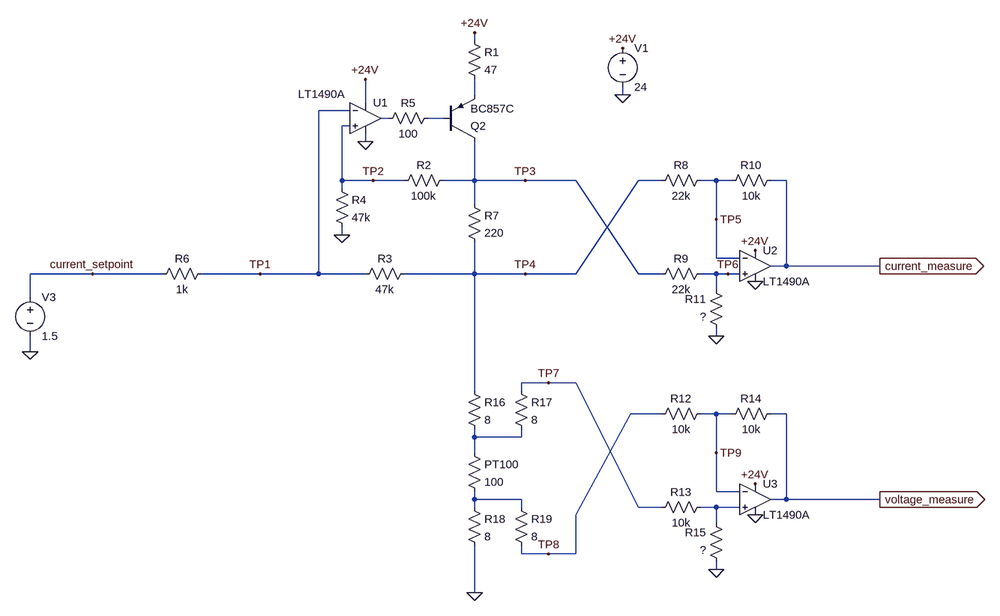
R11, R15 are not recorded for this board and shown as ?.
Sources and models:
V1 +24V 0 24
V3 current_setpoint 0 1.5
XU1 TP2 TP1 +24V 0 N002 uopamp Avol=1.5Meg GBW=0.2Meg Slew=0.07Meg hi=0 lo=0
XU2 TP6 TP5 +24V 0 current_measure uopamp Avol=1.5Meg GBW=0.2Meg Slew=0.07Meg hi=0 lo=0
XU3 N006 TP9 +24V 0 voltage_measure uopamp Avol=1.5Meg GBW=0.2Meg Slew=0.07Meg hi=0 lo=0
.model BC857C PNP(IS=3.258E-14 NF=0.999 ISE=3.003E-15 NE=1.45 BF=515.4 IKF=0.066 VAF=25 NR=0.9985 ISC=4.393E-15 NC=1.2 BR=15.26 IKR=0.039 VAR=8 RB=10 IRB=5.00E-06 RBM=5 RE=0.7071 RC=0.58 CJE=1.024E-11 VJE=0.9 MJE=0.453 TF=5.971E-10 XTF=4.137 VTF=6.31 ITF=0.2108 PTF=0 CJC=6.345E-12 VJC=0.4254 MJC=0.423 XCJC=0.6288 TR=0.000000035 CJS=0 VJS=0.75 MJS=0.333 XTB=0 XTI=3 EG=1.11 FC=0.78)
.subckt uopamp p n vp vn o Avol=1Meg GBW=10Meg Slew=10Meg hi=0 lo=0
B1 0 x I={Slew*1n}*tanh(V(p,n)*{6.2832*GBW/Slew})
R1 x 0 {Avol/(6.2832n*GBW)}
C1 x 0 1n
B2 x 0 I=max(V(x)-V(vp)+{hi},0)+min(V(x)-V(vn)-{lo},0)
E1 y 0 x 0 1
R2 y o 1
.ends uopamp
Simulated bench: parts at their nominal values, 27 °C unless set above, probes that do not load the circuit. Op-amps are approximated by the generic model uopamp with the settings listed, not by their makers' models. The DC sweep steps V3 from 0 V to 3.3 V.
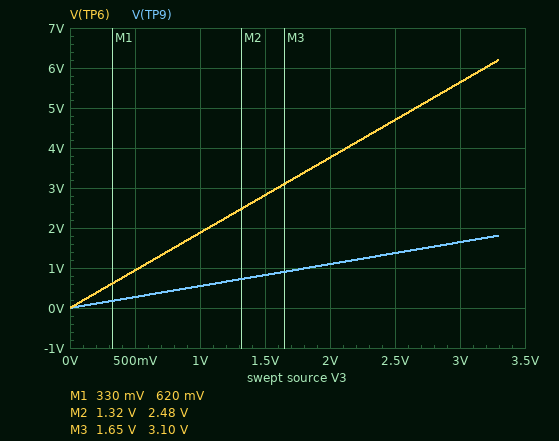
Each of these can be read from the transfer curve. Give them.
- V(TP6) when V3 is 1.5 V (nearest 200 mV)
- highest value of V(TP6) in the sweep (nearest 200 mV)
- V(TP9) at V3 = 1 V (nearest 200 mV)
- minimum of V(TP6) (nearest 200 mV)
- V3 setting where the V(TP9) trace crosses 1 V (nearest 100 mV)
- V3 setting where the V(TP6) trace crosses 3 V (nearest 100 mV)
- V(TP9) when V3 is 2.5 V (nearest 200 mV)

2.8 V
6.2 V
600 mV
0 V
1.8 V
1.6 V
1.4 V
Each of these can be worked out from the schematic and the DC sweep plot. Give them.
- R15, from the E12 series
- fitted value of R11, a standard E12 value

12 kΩ
33 kΩ
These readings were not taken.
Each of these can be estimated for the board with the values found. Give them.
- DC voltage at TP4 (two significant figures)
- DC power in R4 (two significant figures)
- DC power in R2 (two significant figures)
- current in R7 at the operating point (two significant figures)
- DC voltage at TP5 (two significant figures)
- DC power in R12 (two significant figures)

1.6 V
48 µW
100 µW
14 mA
2.8 V
50 µW
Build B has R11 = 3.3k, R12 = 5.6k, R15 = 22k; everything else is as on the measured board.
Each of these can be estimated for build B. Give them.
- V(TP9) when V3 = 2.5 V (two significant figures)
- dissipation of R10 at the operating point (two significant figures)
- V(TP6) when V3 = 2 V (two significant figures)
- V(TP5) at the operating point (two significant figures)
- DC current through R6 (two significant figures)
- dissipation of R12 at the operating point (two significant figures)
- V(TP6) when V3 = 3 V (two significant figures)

1.7 V
21 µW
820 mV
610 mV
2.4 µA
150 µW
1.2 V
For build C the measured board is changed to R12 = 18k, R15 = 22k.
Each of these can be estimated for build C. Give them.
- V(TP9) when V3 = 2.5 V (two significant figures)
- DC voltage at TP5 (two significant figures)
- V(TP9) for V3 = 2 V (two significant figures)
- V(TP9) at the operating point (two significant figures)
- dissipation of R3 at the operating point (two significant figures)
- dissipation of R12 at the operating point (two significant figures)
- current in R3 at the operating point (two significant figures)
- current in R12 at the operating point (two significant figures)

1.7 V
2.8 V
1.4 V
1.0 V
310 nW
48 µW
2.6 µA
51 µA
